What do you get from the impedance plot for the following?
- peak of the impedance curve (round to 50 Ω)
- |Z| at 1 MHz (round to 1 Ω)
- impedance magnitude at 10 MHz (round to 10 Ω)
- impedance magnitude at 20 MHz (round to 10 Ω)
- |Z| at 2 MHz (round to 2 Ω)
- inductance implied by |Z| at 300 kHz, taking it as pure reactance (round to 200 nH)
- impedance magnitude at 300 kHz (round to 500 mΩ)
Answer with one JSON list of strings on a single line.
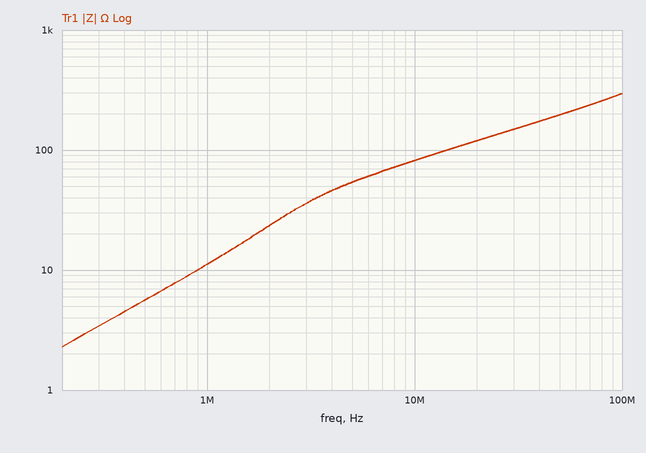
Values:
["300 Ω", "11 Ω", "80 Ω", "120 Ω", "24 Ω", "1.8 µH", "3.5 Ω"]
